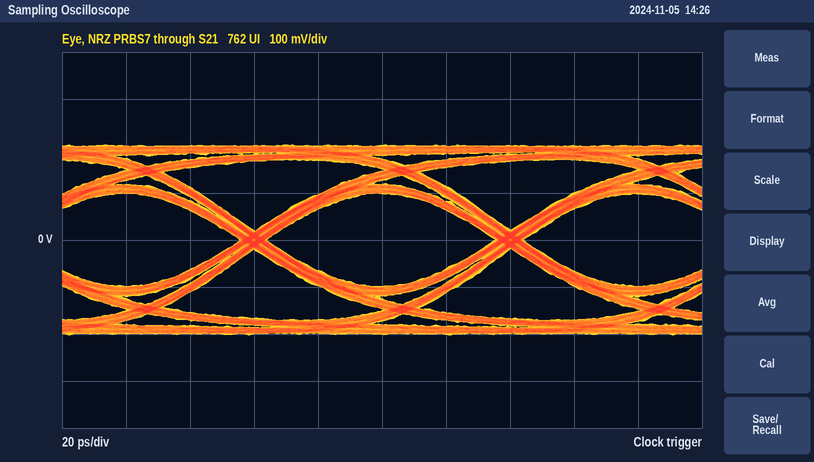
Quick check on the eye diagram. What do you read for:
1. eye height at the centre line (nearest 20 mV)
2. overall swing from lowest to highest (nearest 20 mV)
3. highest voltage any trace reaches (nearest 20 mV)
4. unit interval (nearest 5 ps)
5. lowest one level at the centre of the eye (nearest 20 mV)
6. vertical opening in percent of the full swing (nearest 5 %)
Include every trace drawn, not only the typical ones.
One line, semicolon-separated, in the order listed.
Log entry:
200 mV; 400 mV; 200 mV; 80 ps; 100 mV; 50 %
